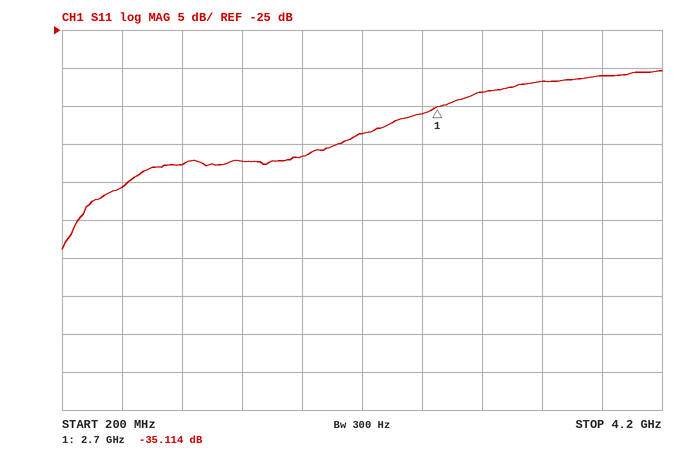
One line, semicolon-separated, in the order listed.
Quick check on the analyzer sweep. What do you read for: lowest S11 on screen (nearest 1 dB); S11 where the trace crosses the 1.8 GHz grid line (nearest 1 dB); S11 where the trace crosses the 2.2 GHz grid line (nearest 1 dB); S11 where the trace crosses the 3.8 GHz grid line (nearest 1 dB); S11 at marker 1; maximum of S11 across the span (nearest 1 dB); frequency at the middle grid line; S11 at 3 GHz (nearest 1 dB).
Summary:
-54 dB; -42 dB; -39 dB; -31 dB; -35.114 dB; -30 dB; 2.2 GHz; -33 dB
